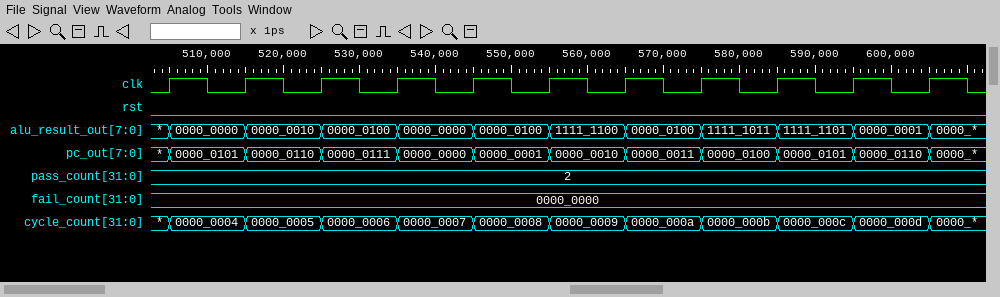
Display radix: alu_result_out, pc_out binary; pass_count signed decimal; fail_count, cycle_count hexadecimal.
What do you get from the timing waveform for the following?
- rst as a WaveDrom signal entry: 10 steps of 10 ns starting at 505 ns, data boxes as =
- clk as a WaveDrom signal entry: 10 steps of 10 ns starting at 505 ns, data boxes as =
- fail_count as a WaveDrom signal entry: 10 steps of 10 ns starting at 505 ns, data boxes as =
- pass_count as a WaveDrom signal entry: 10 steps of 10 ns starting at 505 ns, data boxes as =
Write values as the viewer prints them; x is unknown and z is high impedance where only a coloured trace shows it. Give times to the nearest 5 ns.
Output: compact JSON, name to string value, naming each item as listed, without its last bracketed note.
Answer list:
{"rst as a WaveDrom signal entry: 10 steps of 10 ns starting at 505 ns, data boxes as =": "{name: 'rst', wave: '0.........'}", "clk as a WaveDrom signal entry: 10 steps of 10 ns starting at 505 ns, data boxes as =": "{name: 'clk', wave: 'p.........'}", "fail_count as a WaveDrom signal entry: 10 steps of 10 ns starting at 505 ns, data boxes as =": "{name: 'fail_count', wave: '=.........', data: '0000_0000'}", "pass_count as a WaveDrom signal entry: 10 steps of 10 ns starting at 505 ns, data boxes as =": "{name: 'pass_count', wave: '=.........', data: '2'}"}
